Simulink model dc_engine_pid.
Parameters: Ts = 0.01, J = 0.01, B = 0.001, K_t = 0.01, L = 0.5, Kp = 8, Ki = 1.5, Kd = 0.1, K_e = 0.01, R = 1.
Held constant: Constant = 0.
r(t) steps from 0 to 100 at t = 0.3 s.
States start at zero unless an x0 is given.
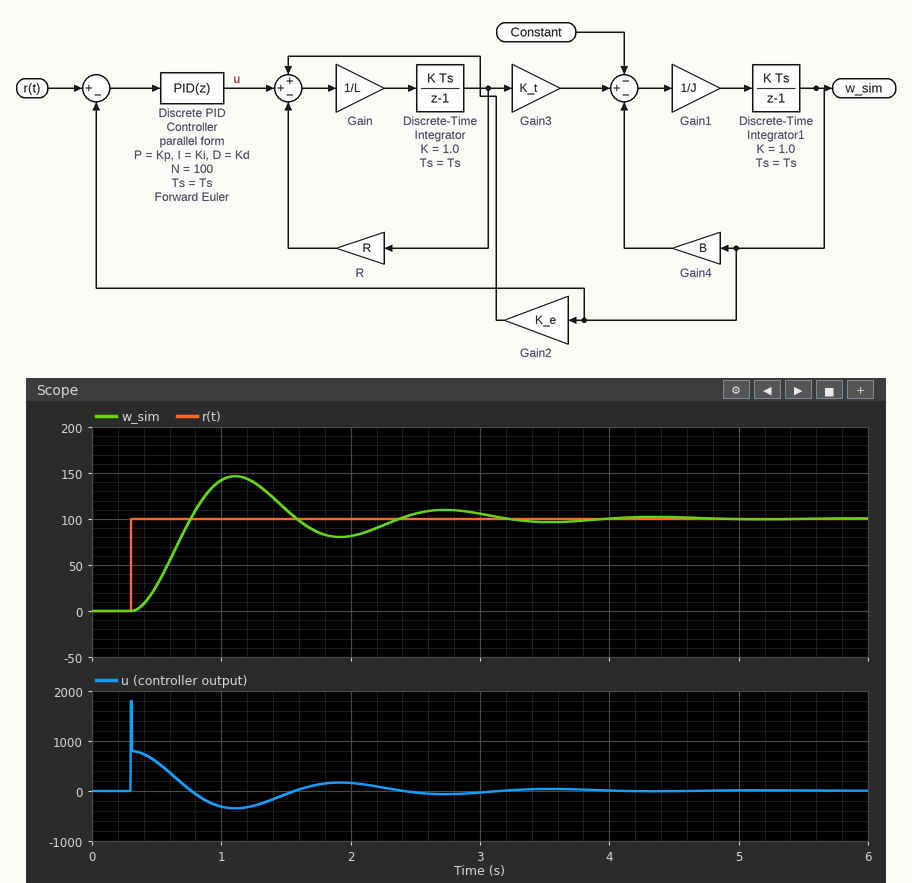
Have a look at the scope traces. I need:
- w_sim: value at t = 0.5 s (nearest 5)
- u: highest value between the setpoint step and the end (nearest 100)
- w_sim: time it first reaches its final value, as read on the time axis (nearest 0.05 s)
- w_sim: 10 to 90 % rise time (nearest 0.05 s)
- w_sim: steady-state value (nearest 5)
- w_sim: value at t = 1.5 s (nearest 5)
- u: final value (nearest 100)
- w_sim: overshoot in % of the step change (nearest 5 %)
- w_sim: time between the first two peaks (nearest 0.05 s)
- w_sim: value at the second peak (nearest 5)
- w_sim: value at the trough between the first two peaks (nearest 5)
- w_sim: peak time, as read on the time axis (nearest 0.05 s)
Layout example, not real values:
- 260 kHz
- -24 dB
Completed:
- 30
- 1800
- 0.75 s
- 0.30 s
- 100
- 110
- 0
- 45 %
- 1.65 s
- 110
- 80
- 1.10 s
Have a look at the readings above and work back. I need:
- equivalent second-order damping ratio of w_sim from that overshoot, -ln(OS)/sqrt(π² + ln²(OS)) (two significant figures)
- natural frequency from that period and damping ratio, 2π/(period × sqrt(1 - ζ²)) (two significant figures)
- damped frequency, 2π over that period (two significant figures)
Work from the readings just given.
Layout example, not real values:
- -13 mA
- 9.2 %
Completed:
- 0.25
- 3.9 rad/s
- 3.8 rad/s
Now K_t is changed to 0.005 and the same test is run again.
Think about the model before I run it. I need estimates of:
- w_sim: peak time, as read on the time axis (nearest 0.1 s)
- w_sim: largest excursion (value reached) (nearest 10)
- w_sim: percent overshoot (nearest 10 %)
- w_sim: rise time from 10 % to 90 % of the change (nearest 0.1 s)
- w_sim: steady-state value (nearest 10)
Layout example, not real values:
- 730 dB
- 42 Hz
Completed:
- 1.5 s
- 130
- 30 %
- 0.5 s
- 100
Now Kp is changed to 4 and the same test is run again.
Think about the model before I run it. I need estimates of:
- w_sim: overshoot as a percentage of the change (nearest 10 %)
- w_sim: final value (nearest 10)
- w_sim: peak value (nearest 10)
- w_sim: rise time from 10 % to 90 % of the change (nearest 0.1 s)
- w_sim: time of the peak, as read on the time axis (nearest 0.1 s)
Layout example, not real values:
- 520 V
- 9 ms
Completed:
- 40 %
- 100
- 140
- 0.5 s
- 1.5 s
